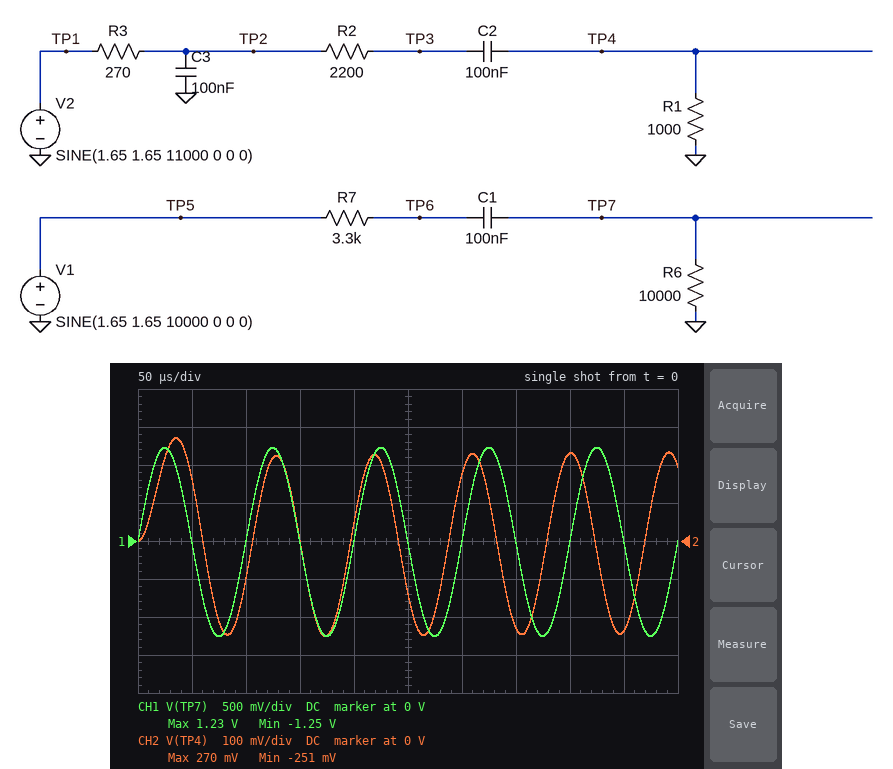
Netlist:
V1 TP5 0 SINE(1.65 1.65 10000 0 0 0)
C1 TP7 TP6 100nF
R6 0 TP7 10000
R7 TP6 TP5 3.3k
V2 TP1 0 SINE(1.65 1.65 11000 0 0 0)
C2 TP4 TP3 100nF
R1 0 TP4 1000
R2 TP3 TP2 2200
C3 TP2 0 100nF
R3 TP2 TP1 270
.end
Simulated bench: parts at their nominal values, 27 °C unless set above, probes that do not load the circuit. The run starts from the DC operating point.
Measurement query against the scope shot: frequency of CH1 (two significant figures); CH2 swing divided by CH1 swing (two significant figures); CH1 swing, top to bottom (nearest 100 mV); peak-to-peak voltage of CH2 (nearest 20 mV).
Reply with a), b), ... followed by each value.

a) 10 kHz
b) 0.21
c) 2.5 V
d) 520 mV
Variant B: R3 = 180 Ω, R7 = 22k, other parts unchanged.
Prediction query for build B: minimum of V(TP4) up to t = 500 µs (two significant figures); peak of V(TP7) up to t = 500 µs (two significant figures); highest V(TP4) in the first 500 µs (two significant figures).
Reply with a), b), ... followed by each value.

a) -330 mV
b) 510 mV
c) 330 mV
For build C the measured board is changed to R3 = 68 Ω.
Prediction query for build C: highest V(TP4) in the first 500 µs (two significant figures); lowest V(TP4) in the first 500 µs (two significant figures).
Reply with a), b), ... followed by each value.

a) 450 mV
b) -480 mV
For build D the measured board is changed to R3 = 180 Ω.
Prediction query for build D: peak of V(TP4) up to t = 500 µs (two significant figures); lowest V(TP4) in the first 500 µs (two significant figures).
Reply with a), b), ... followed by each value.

a) 330 mV
b) -330 mV
